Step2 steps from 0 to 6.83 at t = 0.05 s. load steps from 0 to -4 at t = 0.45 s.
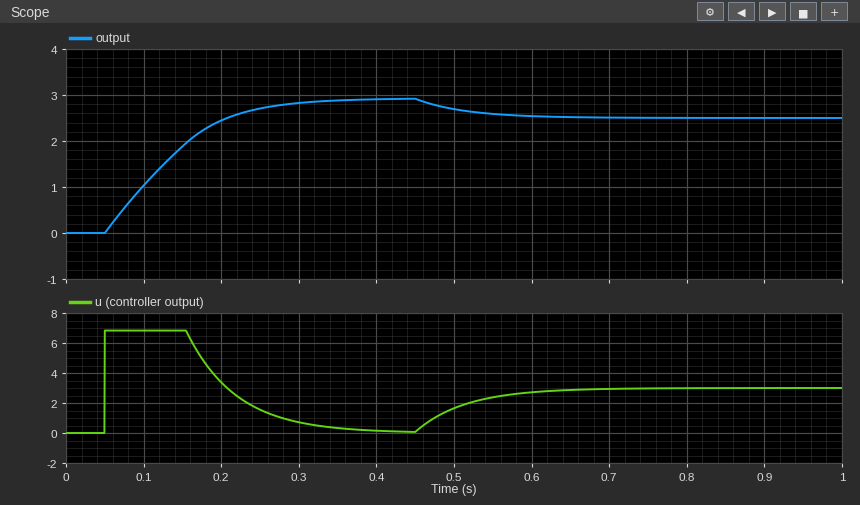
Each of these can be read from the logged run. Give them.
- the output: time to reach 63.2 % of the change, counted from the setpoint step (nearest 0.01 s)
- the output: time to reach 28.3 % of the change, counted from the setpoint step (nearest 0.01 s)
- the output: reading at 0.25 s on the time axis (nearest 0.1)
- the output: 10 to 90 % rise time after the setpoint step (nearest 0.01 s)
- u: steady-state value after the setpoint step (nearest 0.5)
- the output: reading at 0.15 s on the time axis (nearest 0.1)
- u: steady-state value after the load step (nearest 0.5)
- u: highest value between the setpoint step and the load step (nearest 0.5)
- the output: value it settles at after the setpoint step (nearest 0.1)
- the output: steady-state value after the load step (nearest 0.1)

0.10 s
0.04 s
2.7
0.17 s
0.0
1.9
3.0
7.0
2.9
2.5
